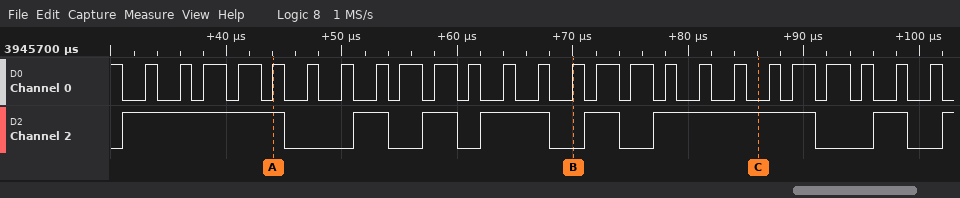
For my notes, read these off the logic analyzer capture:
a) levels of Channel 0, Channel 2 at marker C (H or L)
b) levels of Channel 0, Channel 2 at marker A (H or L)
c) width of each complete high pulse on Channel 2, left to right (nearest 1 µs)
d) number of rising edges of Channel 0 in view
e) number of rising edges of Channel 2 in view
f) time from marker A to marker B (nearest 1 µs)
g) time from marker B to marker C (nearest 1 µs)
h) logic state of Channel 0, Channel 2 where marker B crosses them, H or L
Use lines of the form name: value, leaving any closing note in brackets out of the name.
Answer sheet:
levels of Channel 0, Channel 2 at marker C: Channel 0=L, Channel 2=H
levels of Channel 0, Channel 2 at marker A: Channel 0=H, Channel 2=H
width of each complete high pulse on Channel 2, left to right: 14 µs, 3 µs, 3 µs, 6 µs, 3 µs, 14 µs, 3 µs
number of rising edges of Channel 0 in view: 25
number of rising edges of Channel 2 in view: 8
time from marker A to marker B: 26 µs
time from marker B to marker C: 16 µs
logic state of Channel 0, Channel 2 where marker B crosses them, H or L: Channel 0=H, Channel 2=L
